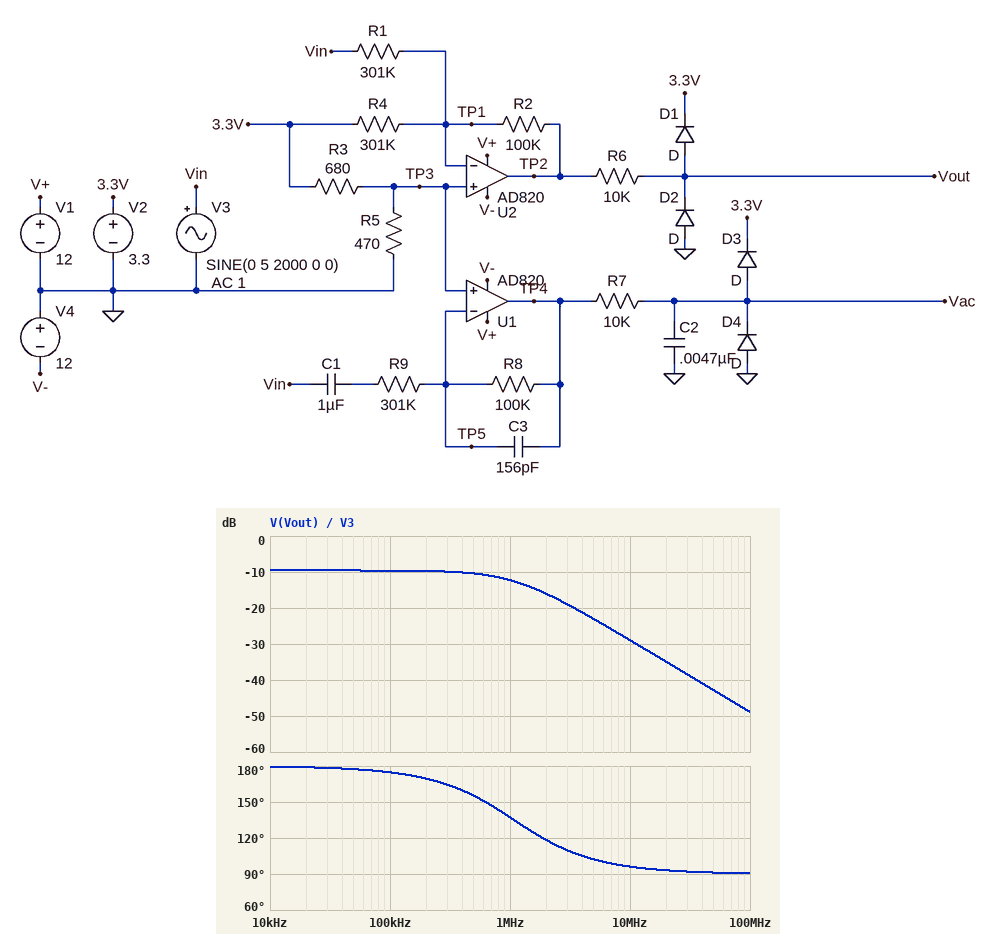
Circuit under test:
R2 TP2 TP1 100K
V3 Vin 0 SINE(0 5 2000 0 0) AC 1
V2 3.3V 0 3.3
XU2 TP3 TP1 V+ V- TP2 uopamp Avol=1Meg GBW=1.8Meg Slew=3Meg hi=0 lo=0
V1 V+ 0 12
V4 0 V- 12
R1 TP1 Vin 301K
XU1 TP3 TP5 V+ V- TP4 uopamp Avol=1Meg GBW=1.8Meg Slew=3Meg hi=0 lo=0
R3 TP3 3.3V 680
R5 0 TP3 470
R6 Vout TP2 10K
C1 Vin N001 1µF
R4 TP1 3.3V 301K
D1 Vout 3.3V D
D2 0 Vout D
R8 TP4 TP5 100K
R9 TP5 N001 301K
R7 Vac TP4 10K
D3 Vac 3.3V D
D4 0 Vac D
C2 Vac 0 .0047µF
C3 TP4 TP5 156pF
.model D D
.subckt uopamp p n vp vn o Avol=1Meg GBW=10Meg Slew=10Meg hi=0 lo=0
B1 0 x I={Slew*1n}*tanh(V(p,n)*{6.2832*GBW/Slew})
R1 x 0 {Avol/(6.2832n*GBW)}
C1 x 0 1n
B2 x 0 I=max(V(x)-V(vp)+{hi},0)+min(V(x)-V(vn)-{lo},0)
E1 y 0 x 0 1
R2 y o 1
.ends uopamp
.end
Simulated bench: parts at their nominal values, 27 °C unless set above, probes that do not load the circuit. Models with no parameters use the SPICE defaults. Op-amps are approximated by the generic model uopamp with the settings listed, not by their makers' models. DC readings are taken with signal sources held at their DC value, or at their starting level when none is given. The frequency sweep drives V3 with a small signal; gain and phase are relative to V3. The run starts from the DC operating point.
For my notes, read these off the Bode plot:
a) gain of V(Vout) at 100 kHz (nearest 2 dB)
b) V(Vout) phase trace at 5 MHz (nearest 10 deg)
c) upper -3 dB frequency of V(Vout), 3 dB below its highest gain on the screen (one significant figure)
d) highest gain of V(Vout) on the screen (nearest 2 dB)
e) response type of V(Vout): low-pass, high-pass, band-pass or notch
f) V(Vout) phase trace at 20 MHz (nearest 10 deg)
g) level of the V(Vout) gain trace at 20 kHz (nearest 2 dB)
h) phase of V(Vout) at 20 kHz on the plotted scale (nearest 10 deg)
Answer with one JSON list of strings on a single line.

["-10 dB", "100 deg", "1 MHz", "-10 dB", "low-pass", "90 deg", "-10 dB", "180 deg"]
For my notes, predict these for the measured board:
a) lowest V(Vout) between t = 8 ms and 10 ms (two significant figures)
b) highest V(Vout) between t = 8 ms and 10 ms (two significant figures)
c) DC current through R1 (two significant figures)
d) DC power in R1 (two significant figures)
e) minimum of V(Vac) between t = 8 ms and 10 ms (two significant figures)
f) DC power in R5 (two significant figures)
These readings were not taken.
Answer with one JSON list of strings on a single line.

["-490 mV", "2.8 V", "4.5 µA", "6.0 µW", "-54 mV", "3.9 mW"]
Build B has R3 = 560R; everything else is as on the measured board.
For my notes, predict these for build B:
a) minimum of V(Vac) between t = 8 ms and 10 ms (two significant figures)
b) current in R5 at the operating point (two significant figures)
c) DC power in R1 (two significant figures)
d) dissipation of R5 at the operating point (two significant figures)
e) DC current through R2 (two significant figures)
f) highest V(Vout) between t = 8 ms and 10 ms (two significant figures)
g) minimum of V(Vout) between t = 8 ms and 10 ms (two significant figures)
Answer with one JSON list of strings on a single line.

["100 mV", "3.2 mA", "7.5 µW", "4.8 mW", "960 nA", "3.1 V", "-250 mV"]
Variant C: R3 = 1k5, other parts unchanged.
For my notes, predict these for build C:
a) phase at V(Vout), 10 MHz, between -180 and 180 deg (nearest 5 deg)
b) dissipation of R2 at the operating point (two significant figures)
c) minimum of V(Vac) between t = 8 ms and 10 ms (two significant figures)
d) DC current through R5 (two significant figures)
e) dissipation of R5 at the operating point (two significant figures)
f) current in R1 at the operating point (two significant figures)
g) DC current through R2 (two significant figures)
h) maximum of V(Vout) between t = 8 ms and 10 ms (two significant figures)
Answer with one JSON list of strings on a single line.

["95 deg", "3.3 µW", "-550 mV", "1.7 mA", "1.3 mW", "2.6 µA", "5.7 µA", "1.9 V"]
